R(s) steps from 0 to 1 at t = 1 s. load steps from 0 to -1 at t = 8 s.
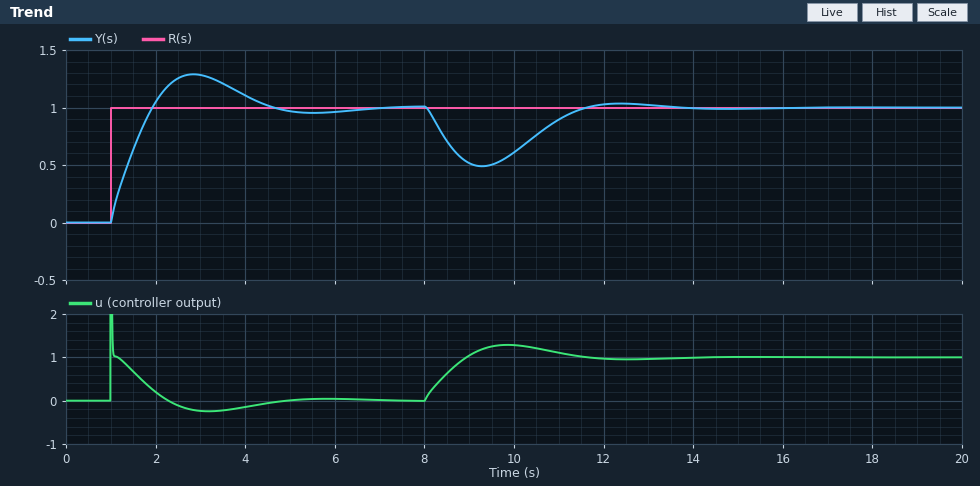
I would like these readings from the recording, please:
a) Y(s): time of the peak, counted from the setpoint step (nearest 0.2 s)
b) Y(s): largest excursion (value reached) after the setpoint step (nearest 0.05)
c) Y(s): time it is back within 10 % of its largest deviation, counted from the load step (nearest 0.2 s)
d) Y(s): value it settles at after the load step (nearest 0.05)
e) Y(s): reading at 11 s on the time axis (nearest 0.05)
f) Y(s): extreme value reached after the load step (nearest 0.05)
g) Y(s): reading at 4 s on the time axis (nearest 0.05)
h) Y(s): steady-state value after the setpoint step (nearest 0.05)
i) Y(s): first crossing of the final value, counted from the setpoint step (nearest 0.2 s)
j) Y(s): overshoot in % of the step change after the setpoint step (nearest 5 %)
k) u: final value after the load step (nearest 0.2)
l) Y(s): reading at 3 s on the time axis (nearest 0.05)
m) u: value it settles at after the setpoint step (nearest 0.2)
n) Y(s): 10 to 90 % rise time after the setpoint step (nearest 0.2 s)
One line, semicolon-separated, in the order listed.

1.8 s; 1.30; 3.2 s; 1.00; 0.90; 0.50; 1.10; 1.00; 1.0 s; 30 %; 1.0; 1.30; 0.0; 0.8 s
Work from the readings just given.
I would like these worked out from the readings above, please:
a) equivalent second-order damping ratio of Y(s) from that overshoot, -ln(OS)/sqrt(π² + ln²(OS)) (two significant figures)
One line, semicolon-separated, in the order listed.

0.36
